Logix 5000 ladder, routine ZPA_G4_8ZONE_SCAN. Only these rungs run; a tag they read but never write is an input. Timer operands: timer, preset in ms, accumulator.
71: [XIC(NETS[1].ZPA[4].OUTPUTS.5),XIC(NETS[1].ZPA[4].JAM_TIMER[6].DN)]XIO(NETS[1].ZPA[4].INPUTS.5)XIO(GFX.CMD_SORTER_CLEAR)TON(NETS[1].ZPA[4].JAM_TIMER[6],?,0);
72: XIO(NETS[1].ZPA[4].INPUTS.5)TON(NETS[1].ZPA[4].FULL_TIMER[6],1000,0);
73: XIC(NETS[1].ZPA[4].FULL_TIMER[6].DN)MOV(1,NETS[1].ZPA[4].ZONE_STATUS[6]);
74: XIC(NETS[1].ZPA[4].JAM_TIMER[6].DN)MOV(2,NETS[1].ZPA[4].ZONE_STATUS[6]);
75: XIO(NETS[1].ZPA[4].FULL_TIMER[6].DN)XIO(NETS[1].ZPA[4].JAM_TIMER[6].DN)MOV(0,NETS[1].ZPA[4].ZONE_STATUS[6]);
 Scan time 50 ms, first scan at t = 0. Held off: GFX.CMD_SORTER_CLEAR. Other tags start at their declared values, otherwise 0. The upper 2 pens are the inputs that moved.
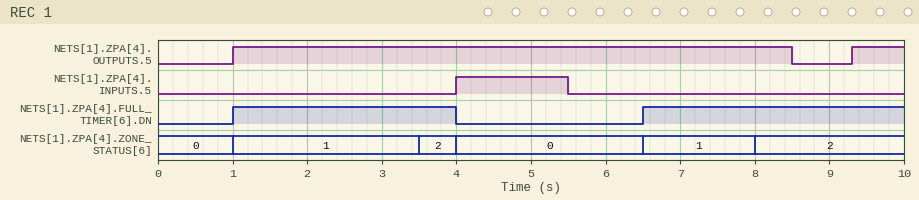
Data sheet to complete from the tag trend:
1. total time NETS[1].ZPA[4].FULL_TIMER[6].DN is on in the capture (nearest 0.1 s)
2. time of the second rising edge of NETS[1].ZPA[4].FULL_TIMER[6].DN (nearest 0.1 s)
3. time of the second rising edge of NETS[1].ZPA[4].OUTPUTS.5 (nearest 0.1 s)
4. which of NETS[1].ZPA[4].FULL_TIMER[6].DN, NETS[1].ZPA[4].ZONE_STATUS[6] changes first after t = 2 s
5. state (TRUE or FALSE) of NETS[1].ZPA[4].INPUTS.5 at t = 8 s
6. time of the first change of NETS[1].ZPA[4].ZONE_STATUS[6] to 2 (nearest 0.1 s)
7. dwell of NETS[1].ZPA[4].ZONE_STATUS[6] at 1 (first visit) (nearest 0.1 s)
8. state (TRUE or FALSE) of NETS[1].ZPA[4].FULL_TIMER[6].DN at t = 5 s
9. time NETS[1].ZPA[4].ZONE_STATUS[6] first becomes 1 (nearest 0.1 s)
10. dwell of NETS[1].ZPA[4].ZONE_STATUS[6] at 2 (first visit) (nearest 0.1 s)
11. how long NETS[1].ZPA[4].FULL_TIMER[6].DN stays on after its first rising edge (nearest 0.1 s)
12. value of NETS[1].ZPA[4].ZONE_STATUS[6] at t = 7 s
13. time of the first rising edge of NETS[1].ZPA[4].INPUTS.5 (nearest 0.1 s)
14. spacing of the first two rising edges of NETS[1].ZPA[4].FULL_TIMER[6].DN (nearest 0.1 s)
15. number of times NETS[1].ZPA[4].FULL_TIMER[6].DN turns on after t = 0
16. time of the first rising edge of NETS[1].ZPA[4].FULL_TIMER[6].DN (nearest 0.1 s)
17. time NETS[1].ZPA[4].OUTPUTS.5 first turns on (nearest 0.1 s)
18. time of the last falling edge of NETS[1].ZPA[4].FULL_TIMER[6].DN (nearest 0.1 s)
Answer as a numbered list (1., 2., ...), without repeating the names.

1. 6.5 s
2. 6.5 s
3. 9.3 s
4. NETS[1].ZPA[4].ZONE_STATUS[6]
5. FALSE
6. 3.5 s
7. 2.5 s
8. FALSE
9. 1.0 s
10. 0.5 s
11. 3.0 s
12. 1
13. 4.0 s
14. 5.5 s
15. 2
16. 1.0 s
17. 1.0 s
18. 4.0 s
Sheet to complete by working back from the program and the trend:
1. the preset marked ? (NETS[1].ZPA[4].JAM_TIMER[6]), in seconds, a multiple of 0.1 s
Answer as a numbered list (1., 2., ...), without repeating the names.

1. 2.5 s
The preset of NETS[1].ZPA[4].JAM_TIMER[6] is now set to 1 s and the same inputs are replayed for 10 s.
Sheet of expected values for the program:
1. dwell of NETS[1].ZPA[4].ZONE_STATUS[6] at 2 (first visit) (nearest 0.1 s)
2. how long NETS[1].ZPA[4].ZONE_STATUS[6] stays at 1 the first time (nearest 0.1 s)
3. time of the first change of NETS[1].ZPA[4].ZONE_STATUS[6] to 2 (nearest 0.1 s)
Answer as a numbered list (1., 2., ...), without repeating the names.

1. 2.0 s
2. 1.0 s
3. 2.0 s
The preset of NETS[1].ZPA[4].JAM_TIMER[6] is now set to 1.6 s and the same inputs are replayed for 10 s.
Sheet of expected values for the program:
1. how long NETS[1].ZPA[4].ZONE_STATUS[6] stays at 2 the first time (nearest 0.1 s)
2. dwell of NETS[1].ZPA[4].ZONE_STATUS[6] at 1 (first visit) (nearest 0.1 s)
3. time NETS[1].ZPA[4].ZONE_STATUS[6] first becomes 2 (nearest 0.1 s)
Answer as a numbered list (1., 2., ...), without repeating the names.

1. 1.4 s
2. 1.6 s
3. 2.6 s
